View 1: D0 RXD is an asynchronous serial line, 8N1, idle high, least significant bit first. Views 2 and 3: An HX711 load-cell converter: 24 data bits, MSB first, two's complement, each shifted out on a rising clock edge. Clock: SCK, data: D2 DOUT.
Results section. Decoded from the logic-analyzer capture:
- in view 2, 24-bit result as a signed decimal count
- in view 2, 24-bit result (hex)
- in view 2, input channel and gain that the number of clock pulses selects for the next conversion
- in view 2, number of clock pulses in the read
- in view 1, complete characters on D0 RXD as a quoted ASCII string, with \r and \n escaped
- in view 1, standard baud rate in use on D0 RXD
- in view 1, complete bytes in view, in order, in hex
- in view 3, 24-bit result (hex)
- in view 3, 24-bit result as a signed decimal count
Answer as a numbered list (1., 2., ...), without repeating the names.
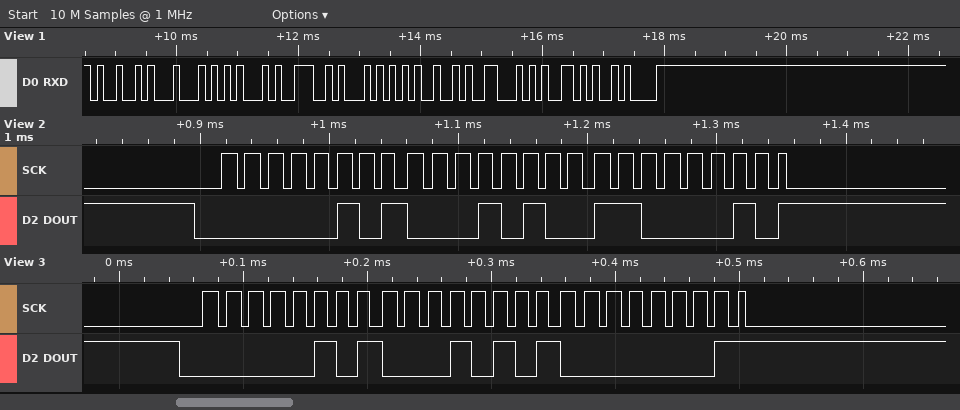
1. 332994
2. 0x0514C2
3. channel A, gain 128
4. 25
5. "IDENTIFY\n"
6. 9600 baud
7. 49 44 45 4E 54 49 46 59 0A
8. 0x051501
9. 333057
